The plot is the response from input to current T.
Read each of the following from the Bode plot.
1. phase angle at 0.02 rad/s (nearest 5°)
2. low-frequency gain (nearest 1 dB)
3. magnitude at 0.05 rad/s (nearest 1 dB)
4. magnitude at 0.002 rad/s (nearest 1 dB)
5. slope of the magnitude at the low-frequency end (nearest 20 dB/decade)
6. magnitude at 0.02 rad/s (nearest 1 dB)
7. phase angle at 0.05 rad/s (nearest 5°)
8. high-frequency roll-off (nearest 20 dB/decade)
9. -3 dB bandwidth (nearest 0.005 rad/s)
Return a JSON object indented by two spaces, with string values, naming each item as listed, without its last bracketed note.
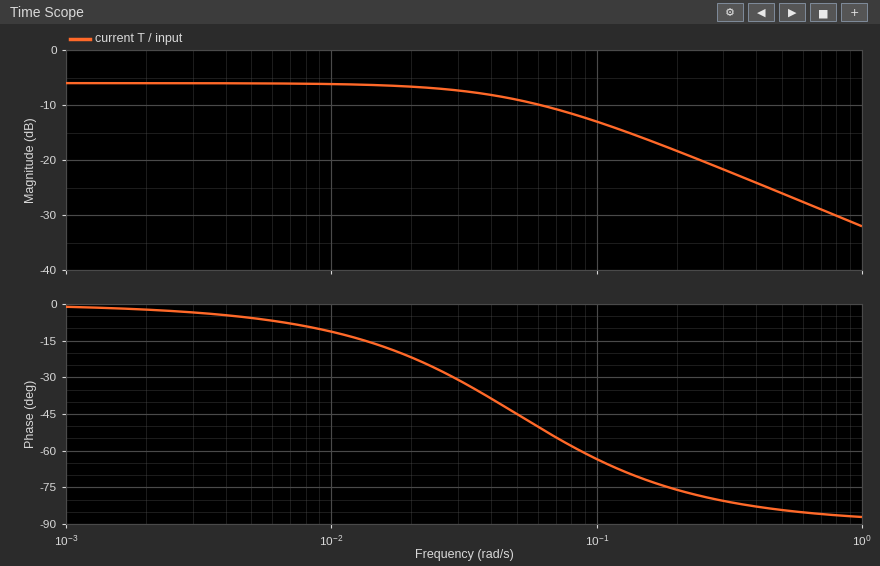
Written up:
{
  "phase angle at 0.02 rad/s": "-20°",
  "low-frequency gain": "-6 dB",
  "magnitude at 0.05 rad/s": "-9 dB",
  "magnitude at 0.002 rad/s": "-6 dB",
  "slope of the magnitude at the low-frequency end": "0 dB/decade",
  "magnitude at 0.02 rad/s": "-7 dB",
  "phase angle at 0.05 rad/s": "-45°",
  "high-frequency roll-off": "-20 dB/decade",
  "-3 dB bandwidth": "0.050 rad/s"
}
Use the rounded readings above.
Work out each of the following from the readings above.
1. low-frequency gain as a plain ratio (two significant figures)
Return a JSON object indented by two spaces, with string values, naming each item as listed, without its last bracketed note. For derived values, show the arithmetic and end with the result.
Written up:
{
  "low-frequency gain as a plain ratio": "10^(-6 / 20) = 0.50"
}
